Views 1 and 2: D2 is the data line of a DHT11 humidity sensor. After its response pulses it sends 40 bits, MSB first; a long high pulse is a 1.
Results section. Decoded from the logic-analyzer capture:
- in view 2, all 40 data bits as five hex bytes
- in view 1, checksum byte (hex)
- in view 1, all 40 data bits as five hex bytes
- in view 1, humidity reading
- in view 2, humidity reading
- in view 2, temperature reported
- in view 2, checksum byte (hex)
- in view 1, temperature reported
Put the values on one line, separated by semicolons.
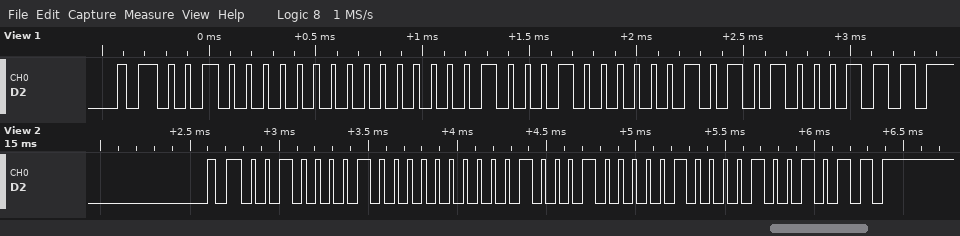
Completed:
21 00 22 08 4B; 0x47; 20 00 22 05 47; 32 %; 33 %; 34.8 °C; 0x4B; 34.5 °C
